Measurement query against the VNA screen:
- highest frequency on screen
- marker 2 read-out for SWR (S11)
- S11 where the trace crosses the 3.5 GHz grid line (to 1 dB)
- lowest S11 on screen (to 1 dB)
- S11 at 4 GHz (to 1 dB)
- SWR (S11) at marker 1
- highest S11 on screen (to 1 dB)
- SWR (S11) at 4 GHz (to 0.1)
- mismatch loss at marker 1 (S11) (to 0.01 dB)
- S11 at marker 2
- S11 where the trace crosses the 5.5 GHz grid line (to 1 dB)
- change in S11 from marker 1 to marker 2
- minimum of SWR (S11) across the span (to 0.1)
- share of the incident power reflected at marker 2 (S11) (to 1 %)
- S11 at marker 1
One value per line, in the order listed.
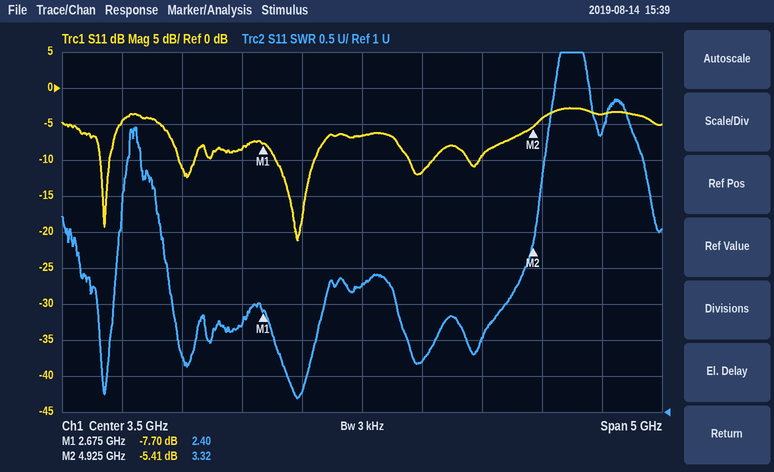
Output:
6 GHz
3.32
-7 dB
-21 dB
-12 dB
2.40
-3 dB
1.7
0.81 dB
-5.41 dB
-4 dB
2.29 dB
1.2
29 %
-7.70 dB
